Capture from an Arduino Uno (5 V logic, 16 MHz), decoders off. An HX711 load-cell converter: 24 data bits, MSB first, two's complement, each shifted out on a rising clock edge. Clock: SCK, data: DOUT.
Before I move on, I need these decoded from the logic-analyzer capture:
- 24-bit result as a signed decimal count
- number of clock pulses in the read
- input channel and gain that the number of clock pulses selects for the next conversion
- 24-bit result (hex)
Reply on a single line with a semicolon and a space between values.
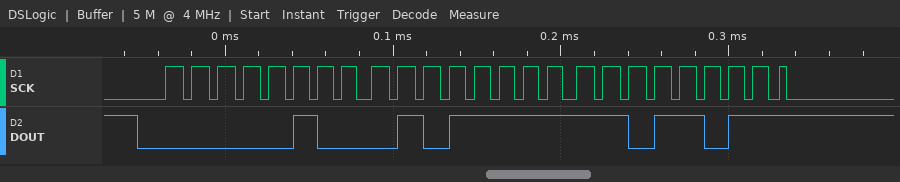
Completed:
286683; 25; channel A, gain 128; 0x045FDB
